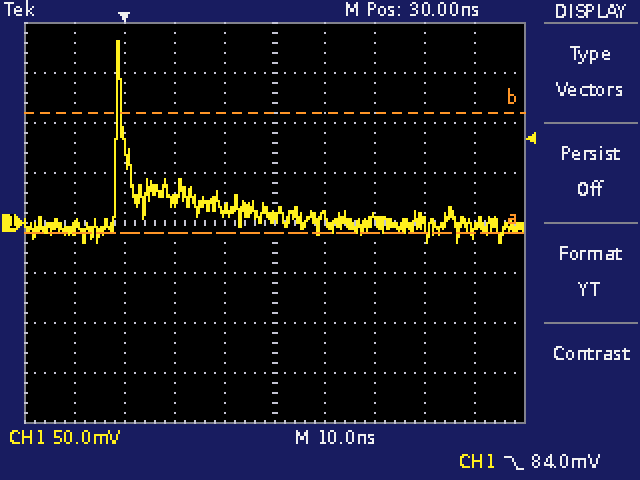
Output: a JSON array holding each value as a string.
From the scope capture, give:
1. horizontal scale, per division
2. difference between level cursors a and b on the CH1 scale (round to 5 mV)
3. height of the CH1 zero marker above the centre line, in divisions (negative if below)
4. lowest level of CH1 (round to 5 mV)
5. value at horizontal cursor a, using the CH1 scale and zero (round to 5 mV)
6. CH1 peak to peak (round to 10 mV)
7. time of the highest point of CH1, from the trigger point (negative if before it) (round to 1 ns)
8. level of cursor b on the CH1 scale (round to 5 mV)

["10 ns", "120 mV", "0.0 div", "-20 mV", "-10 mV", "200 mV", "-1 ns", "110 mV"]
